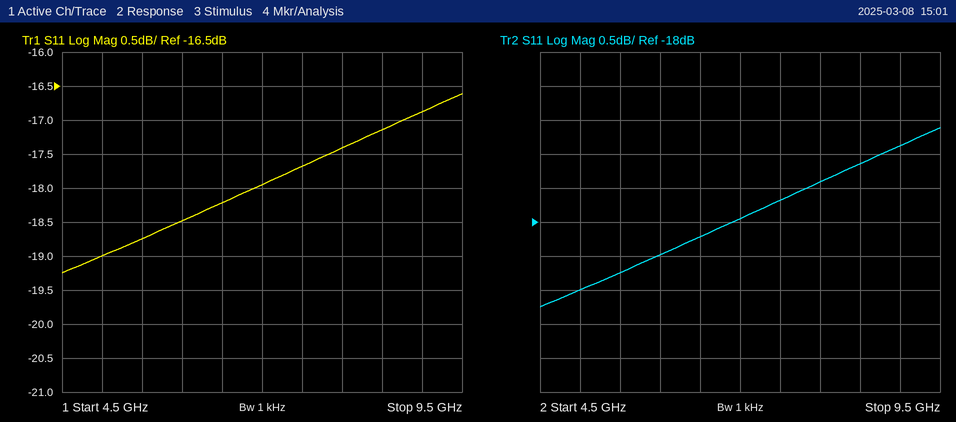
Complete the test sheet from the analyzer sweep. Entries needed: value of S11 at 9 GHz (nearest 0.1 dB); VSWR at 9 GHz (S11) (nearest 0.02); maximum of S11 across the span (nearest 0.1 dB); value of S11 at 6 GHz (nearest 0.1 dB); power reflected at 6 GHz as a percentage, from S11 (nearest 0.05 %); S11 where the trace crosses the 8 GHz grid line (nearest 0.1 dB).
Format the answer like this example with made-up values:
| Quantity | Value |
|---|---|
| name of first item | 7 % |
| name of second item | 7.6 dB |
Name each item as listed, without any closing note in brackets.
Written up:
| Quantity | Value |
|---|---|
| value of S11 at 9 GHz | -16.9 dB |
| VSWR at 9 GHz (S11) | 1.34 |
| maximum of S11 across the span | -16.6 dB |
| value of S11 at 6 GHz | -18.5 dB |
| power reflected at 6 GHz as a percentage, from S11 | 1.40 % |
| S11 where the trace crosses the 8 GHz grid line | -17.4 dB |
